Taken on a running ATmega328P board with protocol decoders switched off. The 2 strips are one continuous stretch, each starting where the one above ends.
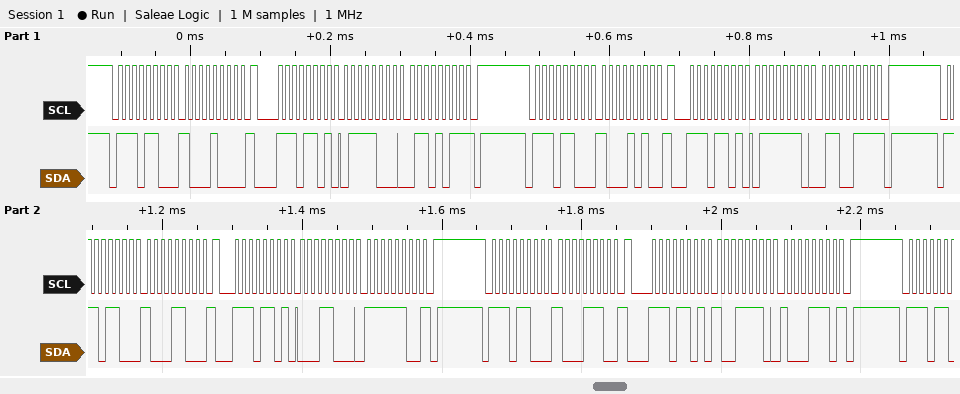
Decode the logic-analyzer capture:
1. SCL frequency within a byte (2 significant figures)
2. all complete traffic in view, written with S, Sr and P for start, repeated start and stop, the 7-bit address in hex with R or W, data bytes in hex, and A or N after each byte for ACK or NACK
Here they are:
100 kHz
S 76W A 88 A Sr 76R A 78 A 6B N P S 76W A 8A A Sr 76R A 7E A 67 N P S 76W A 8C A Sr 76R A 18 A FC N P S 76W A 8E A Sr 76R A 9E A 8E N P
